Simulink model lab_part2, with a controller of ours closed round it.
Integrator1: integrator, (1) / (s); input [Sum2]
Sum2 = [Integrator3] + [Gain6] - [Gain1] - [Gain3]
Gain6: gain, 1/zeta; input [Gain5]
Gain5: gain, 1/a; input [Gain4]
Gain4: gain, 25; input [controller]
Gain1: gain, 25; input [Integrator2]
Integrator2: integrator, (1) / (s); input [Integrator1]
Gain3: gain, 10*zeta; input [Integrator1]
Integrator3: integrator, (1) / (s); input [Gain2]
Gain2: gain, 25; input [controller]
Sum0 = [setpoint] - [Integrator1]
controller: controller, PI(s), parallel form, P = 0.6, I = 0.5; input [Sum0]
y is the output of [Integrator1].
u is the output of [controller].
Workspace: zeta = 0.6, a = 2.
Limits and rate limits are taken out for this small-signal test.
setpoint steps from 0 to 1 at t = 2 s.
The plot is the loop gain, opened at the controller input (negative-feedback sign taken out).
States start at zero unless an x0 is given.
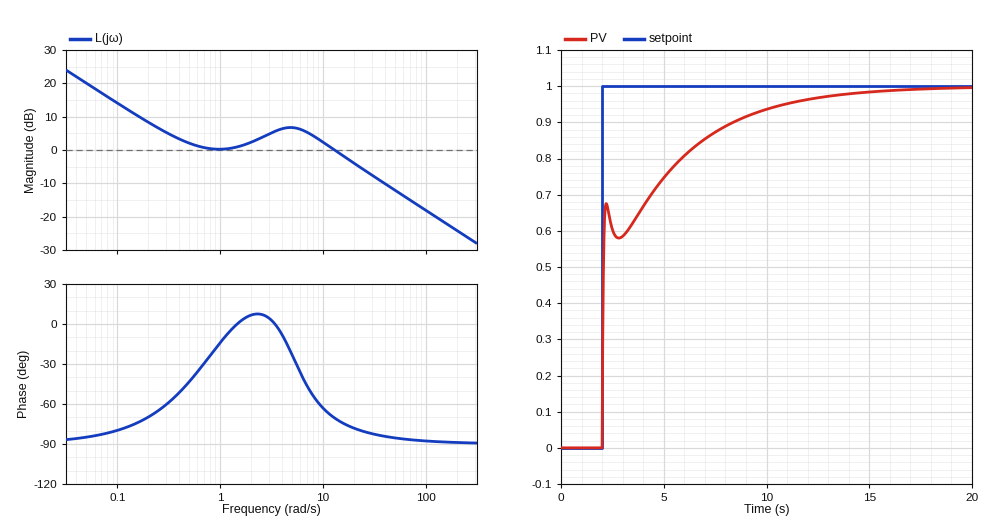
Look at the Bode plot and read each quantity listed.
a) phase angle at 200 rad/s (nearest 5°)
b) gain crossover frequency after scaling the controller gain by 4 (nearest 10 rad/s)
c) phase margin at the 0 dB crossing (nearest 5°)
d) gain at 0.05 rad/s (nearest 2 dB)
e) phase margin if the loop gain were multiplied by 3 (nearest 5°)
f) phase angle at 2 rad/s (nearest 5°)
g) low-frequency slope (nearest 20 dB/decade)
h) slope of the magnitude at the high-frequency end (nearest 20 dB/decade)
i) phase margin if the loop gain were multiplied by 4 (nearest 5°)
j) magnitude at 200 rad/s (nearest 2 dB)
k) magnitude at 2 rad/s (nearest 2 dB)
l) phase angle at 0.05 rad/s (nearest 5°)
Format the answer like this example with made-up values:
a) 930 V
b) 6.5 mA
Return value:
a) -90°
b) 50 rad/s
c) 110°
d) 20 dB
e) 95°
f) 5°
g) -20 dB/decade
h) -20 dB/decade
i) 95°
j) -24 dB
k) 2 dB
l) -85°
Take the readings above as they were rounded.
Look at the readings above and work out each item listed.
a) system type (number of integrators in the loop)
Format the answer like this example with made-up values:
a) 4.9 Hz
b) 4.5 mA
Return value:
a) 1
